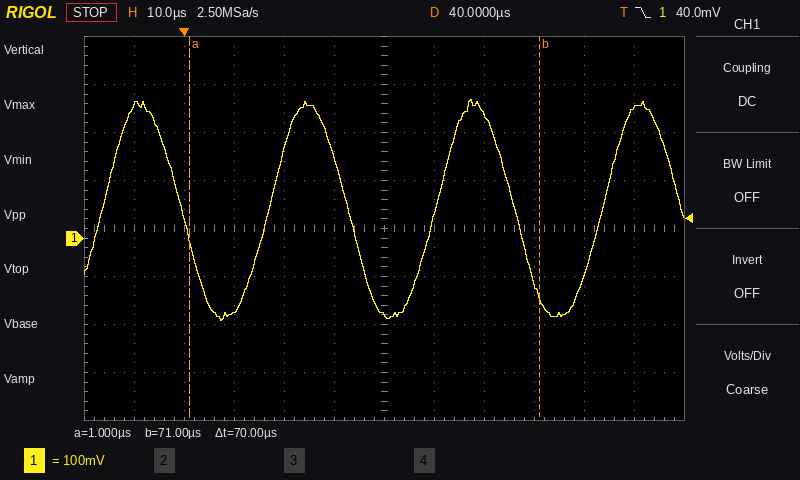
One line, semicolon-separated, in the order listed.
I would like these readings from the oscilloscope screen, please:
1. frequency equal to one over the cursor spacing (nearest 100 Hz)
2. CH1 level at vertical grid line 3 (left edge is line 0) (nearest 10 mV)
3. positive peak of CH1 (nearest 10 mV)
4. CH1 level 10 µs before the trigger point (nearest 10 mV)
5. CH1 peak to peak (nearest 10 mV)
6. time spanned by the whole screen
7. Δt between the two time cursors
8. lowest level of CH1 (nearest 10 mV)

14.3 kHz; -150 mV; 290 mV; 270 mV; 460 mV; 120 µs; 70 µs; -170 mV
